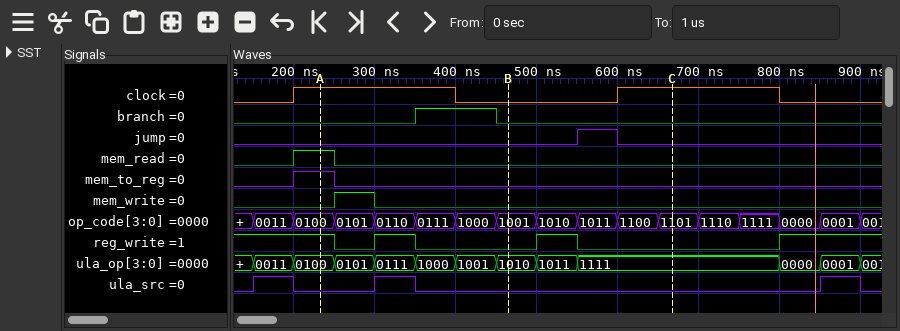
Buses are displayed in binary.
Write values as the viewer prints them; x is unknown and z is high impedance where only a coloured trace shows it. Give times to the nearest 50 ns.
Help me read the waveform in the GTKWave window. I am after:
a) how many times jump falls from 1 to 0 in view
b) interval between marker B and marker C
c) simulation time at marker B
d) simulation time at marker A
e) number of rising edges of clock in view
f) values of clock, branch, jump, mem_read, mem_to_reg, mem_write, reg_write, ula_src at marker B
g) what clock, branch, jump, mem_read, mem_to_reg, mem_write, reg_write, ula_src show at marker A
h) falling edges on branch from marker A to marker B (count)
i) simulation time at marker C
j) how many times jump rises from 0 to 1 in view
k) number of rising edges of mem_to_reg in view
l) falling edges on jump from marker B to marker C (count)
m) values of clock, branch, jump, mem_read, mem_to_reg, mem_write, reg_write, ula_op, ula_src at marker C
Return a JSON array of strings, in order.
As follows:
["1", "200 ns", "450 ns", "250 ns", "2", "clock=0, branch=0, jump=0, mem_read=0, mem_to_reg=0, mem_write=0, reg_write=0, ula_src=0", "clock=1, branch=0, jump=0, mem_read=1, mem_to_reg=1, mem_write=0, reg_write=1, ula_src=0", "1", "650 ns", "1", "1", "1", "clock=1, branch=0, jump=0, mem_read=0, mem_to_reg=0, mem_write=0, reg_write=0, ula_op=1111, ula_src=0"]
